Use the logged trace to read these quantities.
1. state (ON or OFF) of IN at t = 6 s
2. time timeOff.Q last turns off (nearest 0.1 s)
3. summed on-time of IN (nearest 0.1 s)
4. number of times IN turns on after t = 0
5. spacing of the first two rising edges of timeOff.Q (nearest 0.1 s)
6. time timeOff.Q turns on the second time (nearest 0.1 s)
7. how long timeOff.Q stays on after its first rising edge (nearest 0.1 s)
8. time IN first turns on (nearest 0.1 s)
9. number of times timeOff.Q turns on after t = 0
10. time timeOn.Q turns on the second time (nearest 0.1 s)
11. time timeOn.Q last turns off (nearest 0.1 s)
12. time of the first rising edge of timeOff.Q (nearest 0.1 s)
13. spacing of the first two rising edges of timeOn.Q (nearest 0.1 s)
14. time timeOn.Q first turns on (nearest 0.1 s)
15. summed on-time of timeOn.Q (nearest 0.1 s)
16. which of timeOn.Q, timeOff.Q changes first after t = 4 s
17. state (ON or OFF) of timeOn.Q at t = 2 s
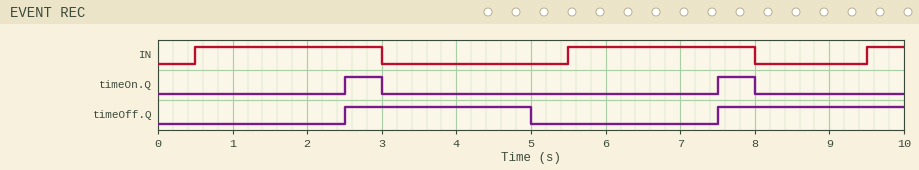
ON
5.0 s
5.5 s
3
5.0 s
7.5 s
2.5 s
0.5 s
2
7.5 s
8.0 s
2.5 s
5.0 s
2.5 s
1.0 s
timeOff.Q
OFF
